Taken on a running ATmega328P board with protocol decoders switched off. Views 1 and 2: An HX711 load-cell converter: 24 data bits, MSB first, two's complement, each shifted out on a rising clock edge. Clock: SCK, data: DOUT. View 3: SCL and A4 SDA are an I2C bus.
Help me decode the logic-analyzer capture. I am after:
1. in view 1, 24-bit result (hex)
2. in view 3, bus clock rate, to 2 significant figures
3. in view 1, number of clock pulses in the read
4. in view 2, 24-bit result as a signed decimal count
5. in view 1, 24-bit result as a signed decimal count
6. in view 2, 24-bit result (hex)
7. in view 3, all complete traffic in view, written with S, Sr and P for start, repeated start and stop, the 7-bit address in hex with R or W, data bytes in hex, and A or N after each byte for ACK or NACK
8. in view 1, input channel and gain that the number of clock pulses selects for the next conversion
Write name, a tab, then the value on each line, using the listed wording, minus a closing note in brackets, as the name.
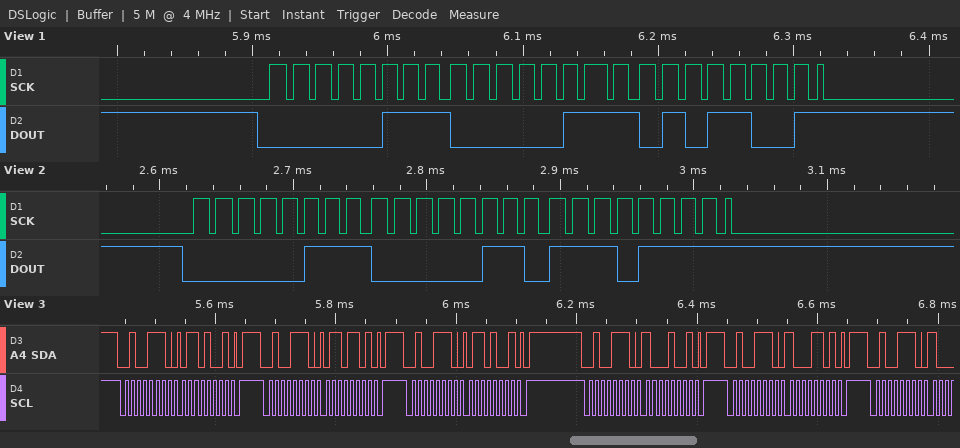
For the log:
in view 1, 24-bit result	0x070759
in view 3, bus clock rate, to 2 significant figures	100 kHz
in view 1, number of clock pulses in the read	25
in view 2, 24-bit result as a signed decimal count	460527
in view 1, 24-bit result as a signed decimal count	460633
in view 2, 24-bit result	0x0706EF
in view 3, all complete traffic in view, written with S, Sr and P for start, repeated start and stop, the 7-bit address in hex with R or W, data bytes in hex, and A or N after each byte for ACK or NACK	S 27W A 69 A P S 27W A 6D A P S 27W A 69 A P S 27W A 89 A P S 27W A 8D A P S 27W A
in view 1, input channel and gain that the number of clock pulses selects for the next conversion	channel A, gain 128
